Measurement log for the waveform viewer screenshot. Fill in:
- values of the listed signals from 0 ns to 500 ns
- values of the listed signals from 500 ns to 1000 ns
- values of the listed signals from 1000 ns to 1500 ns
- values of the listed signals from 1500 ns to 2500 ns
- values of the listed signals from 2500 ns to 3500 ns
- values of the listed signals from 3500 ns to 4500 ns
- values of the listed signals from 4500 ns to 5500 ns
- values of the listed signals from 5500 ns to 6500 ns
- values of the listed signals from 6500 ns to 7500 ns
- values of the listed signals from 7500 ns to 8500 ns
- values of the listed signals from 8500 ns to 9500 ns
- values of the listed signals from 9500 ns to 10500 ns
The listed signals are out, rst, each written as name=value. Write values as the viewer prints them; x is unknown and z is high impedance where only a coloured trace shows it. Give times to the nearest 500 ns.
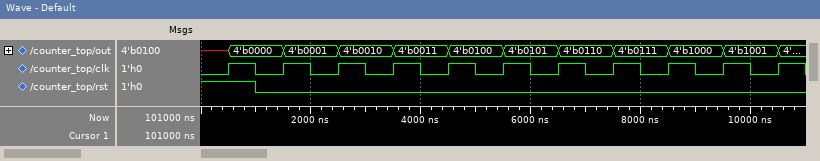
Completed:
out=x, rst=1
out=4'b0000, rst=1
out=4'b0000, rst=0
out=4'b0001, rst=0
out=4'b0010, rst=0
out=4'b0011, rst=0
out=4'b0100, rst=0
out=4'b0101, rst=0
out=4'b0110, rst=0
out=4'b0111, rst=0
out=4'b1000, rst=0
out=4'b1001, rst=0
